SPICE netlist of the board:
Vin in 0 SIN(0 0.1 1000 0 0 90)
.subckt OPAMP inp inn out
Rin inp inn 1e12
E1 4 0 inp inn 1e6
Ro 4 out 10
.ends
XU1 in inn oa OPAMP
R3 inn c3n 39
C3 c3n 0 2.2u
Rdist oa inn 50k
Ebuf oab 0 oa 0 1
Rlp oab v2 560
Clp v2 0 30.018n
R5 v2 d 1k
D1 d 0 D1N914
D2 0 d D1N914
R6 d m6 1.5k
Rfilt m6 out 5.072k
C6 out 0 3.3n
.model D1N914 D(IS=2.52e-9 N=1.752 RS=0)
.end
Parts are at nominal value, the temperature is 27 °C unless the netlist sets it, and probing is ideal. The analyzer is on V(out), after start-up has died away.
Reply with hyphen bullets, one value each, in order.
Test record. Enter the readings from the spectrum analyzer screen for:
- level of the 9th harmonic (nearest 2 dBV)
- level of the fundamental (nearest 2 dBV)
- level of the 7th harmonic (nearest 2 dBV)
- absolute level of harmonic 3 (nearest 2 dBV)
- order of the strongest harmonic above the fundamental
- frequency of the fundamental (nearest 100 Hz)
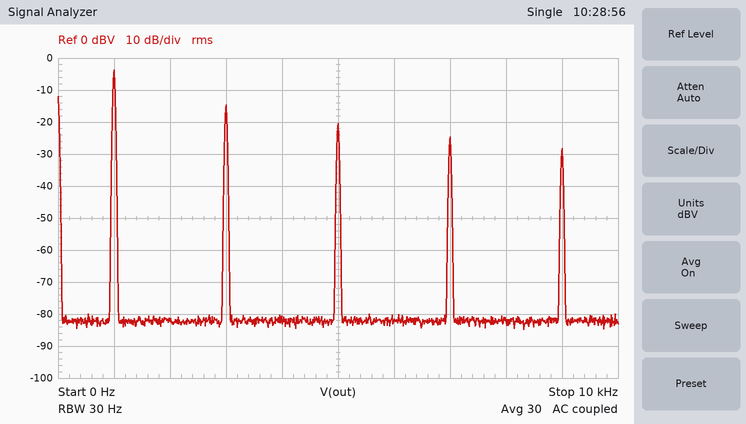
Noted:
- -28 dBV
- -4 dBV
- -24 dBV
- -14 dBV
- 3
- 1.0 kHz
